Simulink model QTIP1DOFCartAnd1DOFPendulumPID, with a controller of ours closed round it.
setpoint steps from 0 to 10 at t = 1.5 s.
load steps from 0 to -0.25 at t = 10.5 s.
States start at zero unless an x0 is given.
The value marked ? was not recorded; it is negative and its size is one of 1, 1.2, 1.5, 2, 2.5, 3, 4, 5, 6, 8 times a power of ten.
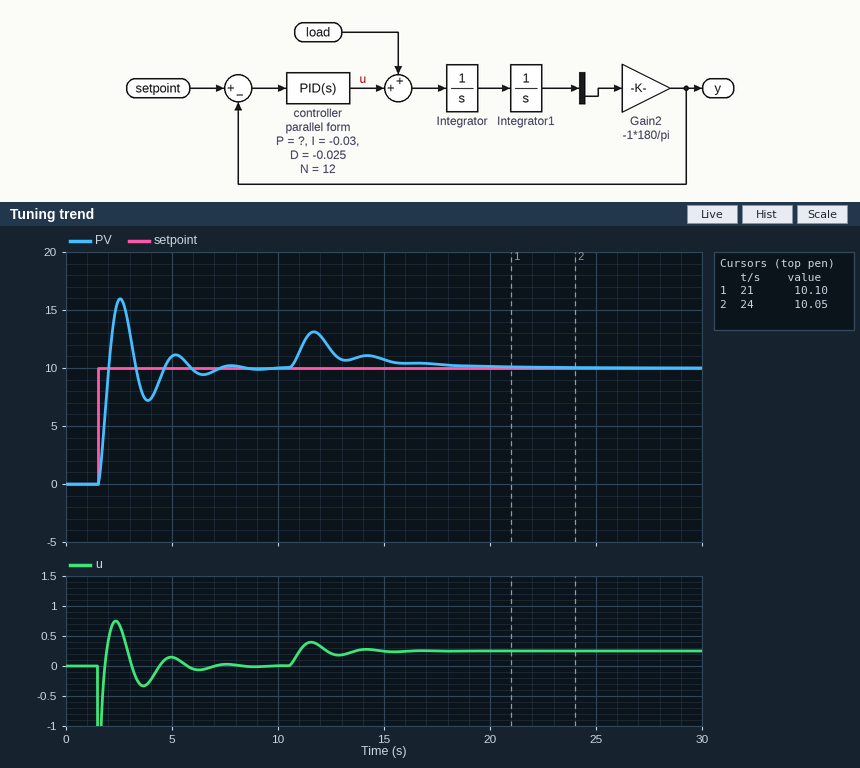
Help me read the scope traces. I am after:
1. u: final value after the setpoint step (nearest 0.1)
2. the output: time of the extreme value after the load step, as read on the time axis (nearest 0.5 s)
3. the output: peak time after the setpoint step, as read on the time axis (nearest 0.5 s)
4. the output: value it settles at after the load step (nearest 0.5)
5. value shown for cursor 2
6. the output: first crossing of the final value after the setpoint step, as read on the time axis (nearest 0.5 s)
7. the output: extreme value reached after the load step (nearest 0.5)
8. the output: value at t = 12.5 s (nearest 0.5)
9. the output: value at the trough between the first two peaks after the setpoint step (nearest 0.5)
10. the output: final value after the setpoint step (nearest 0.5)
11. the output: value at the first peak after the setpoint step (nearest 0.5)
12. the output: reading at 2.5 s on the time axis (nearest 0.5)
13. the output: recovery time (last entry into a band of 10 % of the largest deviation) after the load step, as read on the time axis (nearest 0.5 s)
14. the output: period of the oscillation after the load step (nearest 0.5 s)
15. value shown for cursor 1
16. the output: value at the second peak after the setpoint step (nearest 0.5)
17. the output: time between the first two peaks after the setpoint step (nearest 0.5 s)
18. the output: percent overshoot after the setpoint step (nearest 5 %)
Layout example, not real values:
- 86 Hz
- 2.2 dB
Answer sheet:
- 0.0
- 11.5 s
- 2.5 s
- 10.0
- 10.05
- 2.0 s
- 13.0
- 11.5
- 7.0
- 10.0
- 16.0
- 16.0
- 17.5 s
- 2.5 s
- 10.10
- 11.0
- 2.5 s
- 60 %
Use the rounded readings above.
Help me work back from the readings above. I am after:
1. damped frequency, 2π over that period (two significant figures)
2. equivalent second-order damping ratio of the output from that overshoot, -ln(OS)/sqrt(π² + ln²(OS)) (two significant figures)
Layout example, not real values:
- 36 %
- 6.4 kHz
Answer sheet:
- 2.5 rad/s
- 0.16
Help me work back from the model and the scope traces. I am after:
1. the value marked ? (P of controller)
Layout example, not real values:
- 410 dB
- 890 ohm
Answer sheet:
- -0.1
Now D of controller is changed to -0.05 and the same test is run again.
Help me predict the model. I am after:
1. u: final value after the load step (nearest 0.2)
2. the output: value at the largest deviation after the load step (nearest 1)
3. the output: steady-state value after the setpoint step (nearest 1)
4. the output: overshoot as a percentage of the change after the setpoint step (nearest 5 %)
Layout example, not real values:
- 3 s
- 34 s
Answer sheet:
- 0.2
- 12
- 10
- 35 %
